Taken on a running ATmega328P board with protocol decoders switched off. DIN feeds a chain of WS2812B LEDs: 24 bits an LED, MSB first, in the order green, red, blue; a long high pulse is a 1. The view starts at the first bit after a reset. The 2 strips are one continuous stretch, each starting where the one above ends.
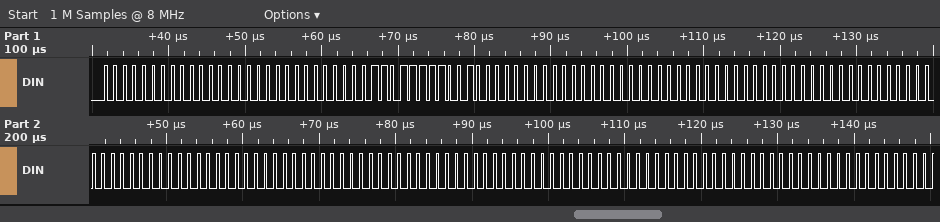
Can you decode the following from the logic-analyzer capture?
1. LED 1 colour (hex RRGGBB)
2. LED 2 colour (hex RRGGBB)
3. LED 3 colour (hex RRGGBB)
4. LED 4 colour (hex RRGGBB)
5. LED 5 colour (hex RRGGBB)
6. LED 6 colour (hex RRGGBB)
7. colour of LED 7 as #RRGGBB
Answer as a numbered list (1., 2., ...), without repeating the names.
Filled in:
1. #000000
2. #F20D00
3. #000000
4. #000000
5. #000000
6. #000000
7. #000000
